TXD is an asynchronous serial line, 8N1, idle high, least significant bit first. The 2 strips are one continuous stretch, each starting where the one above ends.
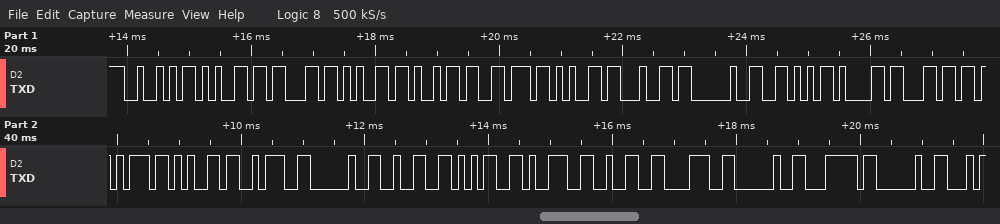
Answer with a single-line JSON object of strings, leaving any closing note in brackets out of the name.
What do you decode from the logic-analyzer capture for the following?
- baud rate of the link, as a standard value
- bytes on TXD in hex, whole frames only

{"baud rate of the link, as a standard value": "9600 baud", "bytes on TXD in hex, whole frames only": "52 65 63 65 69 76 65 64 20 56 61 6C 75 65 3A 20 32 35 39 32 38 20 7C 20"}
